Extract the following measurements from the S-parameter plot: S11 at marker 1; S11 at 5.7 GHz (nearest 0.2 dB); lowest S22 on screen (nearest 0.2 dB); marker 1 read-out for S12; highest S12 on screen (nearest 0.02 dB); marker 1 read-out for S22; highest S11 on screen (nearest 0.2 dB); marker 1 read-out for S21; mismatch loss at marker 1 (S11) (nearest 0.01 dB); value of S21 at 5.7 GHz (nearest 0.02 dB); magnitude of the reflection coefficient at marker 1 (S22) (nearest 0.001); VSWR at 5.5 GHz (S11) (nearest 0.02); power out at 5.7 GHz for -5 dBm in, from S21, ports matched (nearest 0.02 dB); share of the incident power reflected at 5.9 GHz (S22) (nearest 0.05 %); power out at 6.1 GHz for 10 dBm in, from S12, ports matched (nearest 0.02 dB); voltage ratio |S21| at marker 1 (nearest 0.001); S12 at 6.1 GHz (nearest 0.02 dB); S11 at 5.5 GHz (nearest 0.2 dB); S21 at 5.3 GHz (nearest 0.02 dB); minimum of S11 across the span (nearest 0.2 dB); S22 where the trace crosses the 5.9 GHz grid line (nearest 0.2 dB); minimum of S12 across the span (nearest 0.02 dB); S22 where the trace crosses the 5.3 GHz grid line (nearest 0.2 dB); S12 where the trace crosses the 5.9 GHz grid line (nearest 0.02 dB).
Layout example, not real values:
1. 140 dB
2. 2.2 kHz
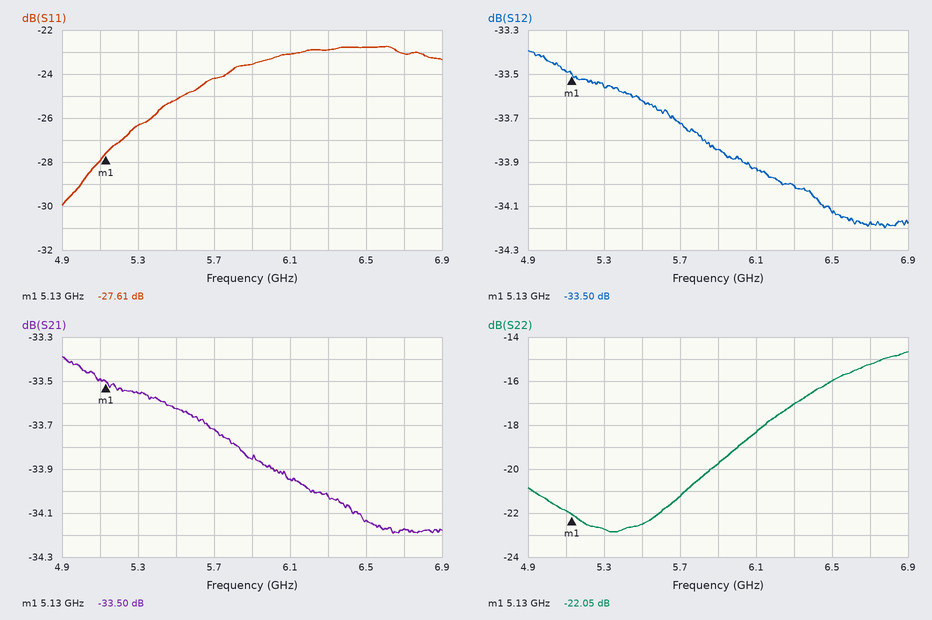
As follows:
1. -27.61 dB
2. -24.2 dB
3. -22.8 dB
4. -33.50 dB
5. -33.40 dB
6. -22.05 dB
7. -22.8 dB
8. -33.50 dB
9. 0.01 dB
10. -33.72 dB
11. 0.079
12. 1.12
13. -38.72 dBm
14. 1.05 %
15. -23.92 dBm
16. 0.021
17. -33.92 dB
18. -25.2 dB
19. -33.56 dB
20. -30.0 dB
21. -19.8 dB
22. -34.20 dB
23. -22.8 dB
24. -33.84 dB
